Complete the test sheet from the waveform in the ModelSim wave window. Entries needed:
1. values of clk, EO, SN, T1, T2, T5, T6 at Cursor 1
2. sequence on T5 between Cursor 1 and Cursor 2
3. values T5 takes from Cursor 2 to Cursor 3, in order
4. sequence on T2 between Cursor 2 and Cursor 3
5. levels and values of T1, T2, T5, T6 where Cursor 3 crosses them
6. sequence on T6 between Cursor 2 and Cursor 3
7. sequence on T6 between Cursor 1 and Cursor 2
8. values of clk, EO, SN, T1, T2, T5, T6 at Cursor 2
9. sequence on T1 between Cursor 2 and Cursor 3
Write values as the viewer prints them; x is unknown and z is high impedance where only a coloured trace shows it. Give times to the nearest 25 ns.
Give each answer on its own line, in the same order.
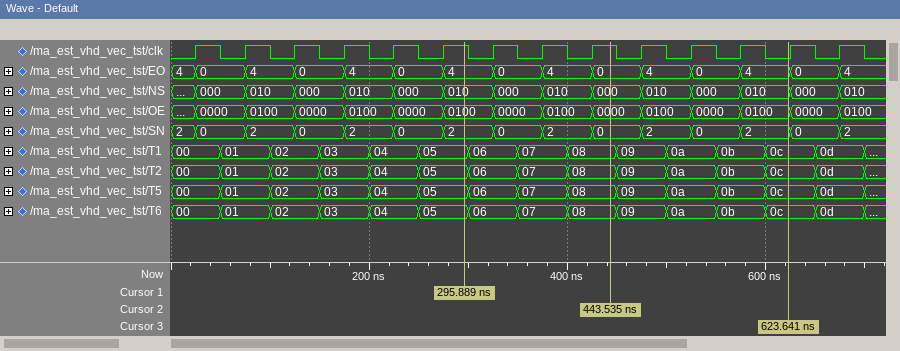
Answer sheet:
clk=1, EO=4, SN=2, T1=05, T2=05, T5=05, T6=05
05, 06, 07, 08
08, 09, 0a, 0b, 0c
08, 09, 0a, 0b, 0c
T1=0c, T2=0c, T5=0c, T6=0c
08, 09, 0a, 0b, 0c
05, 06, 07, 08
clk=1, EO=0, SN=0, T1=08, T2=08, T5=08, T6=08
08, 09, 0a, 0b, 0c
